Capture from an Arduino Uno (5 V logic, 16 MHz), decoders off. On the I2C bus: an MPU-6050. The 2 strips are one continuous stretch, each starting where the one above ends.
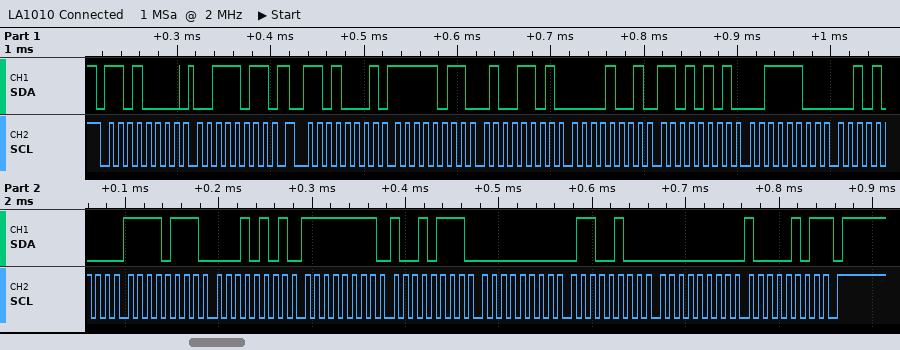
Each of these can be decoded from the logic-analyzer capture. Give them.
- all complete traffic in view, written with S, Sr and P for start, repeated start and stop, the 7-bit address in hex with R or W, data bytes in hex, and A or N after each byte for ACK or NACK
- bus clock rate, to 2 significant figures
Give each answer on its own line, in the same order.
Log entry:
S 68W A 3B A Sr 68R A FB A 4D A 09 A D5 A 3C A 28 A F7 A 15 A FF A 97 A 00 A 64 A 00 A 85 N P
100 kHz
